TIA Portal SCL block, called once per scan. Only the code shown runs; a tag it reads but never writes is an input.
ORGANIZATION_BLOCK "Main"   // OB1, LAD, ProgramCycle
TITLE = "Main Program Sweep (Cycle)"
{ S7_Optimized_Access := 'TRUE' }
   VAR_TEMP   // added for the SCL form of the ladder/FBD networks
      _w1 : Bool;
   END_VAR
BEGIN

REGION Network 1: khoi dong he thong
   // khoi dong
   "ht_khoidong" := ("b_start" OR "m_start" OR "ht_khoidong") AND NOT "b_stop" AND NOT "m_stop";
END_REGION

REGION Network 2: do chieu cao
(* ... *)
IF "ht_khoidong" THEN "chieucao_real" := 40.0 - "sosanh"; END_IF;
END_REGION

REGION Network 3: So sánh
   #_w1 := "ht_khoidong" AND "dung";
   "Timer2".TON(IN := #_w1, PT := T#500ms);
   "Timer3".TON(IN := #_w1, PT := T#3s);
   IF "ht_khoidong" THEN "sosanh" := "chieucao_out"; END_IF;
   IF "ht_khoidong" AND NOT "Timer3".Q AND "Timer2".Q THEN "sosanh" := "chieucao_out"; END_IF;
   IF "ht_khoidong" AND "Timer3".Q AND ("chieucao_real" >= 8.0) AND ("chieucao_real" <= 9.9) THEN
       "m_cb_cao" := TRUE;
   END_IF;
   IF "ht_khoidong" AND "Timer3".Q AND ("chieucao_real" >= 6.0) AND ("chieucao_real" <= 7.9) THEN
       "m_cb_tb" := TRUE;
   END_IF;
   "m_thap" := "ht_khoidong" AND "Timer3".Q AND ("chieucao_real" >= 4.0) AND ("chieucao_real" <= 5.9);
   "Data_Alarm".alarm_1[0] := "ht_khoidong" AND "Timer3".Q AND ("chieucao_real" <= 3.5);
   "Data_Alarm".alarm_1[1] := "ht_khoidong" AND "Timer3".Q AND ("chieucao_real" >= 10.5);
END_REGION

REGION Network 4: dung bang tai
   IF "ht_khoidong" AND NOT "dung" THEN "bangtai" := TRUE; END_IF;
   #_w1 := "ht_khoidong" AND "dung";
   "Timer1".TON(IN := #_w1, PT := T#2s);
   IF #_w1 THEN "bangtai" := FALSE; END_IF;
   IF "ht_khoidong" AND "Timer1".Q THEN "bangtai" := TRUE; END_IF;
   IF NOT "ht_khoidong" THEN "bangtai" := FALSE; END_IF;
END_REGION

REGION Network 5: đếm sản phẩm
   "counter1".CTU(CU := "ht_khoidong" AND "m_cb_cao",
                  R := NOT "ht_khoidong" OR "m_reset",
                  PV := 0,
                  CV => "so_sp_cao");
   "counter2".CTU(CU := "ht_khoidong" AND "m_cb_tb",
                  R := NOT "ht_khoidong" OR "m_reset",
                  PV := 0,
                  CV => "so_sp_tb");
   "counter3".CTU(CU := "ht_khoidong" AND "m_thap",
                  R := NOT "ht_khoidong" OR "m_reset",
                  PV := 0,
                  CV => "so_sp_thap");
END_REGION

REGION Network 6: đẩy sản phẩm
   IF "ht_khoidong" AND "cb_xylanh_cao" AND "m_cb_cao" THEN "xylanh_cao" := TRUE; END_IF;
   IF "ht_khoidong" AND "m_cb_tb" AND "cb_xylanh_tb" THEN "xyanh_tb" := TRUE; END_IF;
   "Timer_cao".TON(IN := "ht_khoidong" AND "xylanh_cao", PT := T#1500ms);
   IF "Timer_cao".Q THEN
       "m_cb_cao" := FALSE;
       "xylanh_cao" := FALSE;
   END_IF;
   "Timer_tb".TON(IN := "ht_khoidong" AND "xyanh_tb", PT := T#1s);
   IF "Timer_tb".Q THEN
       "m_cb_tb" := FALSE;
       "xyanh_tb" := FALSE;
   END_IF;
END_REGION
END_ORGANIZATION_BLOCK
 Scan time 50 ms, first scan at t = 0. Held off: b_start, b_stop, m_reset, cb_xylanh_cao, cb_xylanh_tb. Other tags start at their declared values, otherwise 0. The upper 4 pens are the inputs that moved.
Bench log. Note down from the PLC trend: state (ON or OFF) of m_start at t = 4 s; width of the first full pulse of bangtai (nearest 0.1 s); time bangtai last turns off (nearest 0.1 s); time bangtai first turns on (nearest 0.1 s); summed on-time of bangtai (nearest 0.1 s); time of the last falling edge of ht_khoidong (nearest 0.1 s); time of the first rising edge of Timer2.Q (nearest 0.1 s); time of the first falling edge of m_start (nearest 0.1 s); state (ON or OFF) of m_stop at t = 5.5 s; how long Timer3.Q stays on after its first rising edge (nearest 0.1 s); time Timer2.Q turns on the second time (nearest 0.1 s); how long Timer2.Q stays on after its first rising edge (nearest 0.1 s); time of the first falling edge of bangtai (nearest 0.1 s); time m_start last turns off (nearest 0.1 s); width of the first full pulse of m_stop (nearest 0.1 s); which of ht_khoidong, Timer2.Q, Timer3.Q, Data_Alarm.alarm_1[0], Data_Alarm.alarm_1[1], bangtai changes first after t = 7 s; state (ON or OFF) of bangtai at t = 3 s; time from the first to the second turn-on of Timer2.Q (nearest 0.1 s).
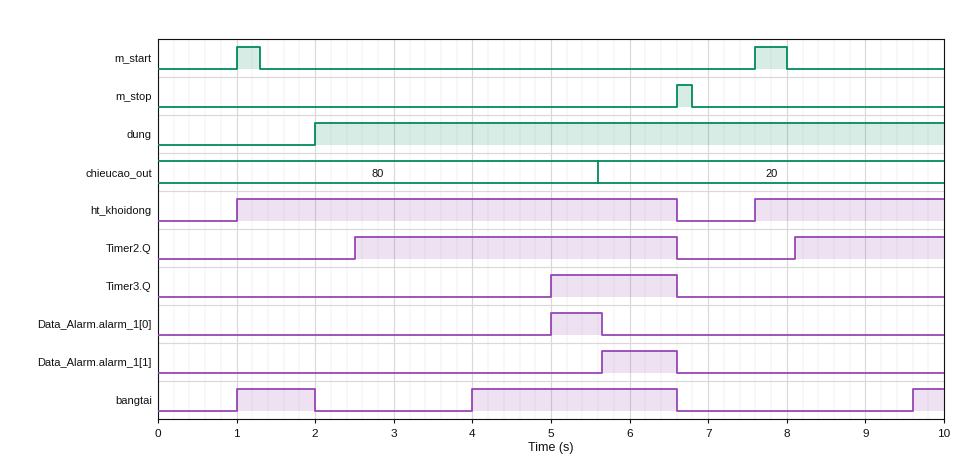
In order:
OFF
1.0 s
6.6 s
1.0 s
4.0 s
6.6 s
2.5 s
1.3 s
OFF
1.6 s
8.1 s
4.1 s
2.0 s
8.0 s
0.2 s
ht_khoidong
OFF
5.6 s
